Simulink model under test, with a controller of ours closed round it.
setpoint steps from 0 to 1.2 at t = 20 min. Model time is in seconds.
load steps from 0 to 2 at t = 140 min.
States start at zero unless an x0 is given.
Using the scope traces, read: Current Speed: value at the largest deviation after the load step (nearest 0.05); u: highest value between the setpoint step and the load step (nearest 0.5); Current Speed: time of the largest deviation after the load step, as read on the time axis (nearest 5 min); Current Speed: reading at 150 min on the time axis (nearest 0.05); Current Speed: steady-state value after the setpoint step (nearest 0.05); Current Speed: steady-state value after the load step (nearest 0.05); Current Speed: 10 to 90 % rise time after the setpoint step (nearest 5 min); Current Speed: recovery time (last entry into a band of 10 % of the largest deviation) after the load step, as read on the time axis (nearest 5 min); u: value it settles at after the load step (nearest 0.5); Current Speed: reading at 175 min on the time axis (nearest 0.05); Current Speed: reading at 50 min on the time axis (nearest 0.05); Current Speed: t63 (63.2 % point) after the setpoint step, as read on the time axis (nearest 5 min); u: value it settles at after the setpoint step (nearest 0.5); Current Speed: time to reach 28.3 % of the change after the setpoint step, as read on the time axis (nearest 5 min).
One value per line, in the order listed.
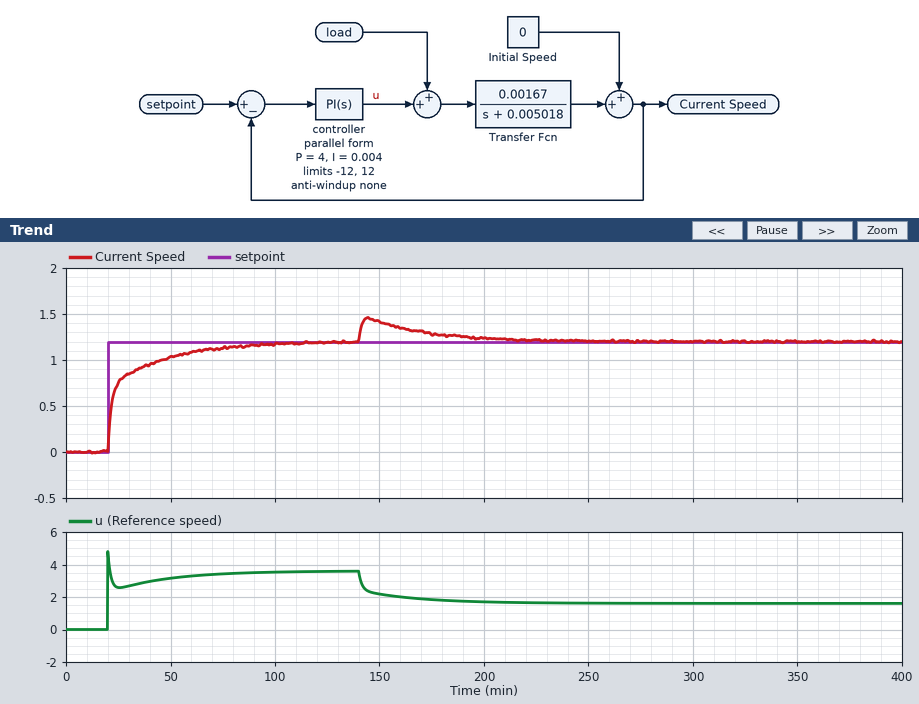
1.45
5.0
145 min
1.40
1.20
1.20
40 min
210 min
1.5
1.30
1.05
25 min
3.5
20 min
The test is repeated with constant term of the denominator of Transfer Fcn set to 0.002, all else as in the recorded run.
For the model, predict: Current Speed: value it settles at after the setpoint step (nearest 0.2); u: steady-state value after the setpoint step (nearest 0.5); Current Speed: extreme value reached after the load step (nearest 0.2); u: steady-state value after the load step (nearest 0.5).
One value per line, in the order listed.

1.2
1.5
1.6
-0.5
